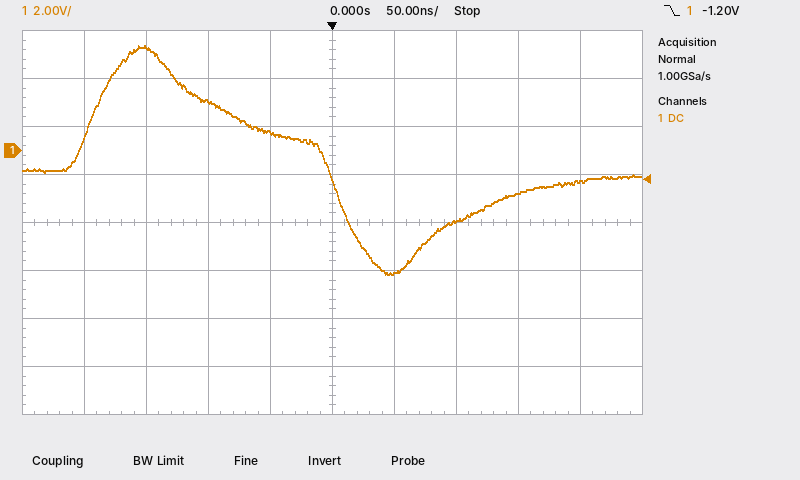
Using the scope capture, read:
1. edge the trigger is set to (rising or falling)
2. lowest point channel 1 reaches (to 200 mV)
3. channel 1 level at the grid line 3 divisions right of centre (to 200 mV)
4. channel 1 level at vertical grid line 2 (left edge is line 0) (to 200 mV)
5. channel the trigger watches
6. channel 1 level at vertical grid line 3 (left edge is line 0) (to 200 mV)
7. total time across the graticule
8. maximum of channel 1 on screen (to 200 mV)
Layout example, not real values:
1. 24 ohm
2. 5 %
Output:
1. falling
2. -5.2 V
3. -1.8 V
4. 4.2 V
5. channel 1
6. 2.0 V
7. 500 ns
8. 4.4 V
